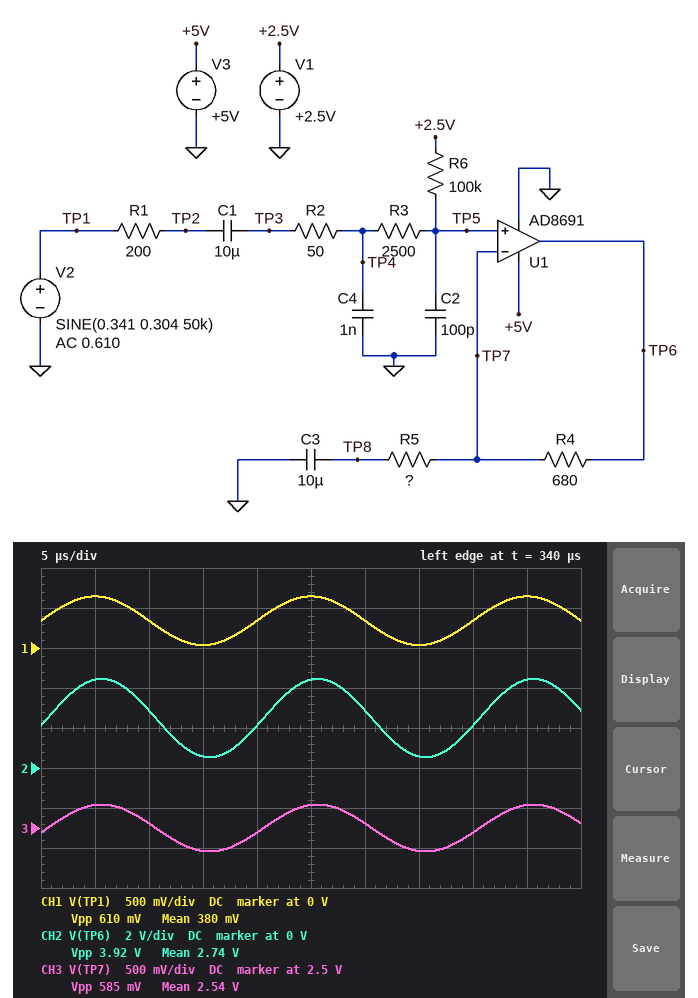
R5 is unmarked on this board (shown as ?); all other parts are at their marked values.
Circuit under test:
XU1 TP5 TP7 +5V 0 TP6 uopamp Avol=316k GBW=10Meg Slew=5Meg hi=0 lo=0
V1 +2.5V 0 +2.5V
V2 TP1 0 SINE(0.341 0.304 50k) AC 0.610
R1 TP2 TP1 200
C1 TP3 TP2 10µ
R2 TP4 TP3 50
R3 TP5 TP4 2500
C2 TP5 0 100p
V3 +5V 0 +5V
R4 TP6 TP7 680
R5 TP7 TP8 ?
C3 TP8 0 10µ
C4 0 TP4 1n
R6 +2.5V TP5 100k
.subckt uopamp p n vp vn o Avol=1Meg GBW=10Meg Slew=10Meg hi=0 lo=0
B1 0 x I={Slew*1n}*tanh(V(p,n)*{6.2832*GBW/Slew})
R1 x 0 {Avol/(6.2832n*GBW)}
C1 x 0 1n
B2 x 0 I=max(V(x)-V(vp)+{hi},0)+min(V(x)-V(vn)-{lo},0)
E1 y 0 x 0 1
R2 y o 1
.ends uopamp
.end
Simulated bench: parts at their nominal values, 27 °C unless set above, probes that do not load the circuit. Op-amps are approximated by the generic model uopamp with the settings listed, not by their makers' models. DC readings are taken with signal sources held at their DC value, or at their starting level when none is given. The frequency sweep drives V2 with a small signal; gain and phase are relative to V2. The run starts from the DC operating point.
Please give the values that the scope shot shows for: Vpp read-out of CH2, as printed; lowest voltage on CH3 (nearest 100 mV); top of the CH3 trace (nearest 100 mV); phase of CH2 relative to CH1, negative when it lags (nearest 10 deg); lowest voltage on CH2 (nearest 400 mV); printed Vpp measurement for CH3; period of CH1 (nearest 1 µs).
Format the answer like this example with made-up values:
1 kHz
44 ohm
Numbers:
3.92 V
2.2 V
2.8 V
-10 deg
400 mV
585 mV
20 µs
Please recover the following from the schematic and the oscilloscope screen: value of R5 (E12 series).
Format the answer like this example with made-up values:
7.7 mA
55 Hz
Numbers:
120 Ω
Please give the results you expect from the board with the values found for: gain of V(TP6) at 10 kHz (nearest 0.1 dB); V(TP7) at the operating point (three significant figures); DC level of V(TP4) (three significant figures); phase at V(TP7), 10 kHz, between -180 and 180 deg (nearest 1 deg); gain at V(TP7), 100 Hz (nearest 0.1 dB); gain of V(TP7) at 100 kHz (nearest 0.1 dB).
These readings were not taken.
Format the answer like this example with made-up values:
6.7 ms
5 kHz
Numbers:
16.2 dB
2.50 V
2.50 V
-2 deg
-0.2 dB
-0.5 dB
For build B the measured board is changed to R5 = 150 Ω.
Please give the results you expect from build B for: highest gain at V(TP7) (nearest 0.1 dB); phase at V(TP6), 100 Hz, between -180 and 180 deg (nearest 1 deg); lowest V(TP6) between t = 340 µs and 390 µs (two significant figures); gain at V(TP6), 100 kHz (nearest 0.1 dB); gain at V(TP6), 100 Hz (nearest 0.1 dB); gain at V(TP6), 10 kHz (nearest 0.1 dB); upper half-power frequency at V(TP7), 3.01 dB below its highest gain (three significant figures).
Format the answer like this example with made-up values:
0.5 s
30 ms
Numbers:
-0.2 dB
36 deg
870 mV
14.4 dB
11.5 dB
14.6 dB
374 kHz
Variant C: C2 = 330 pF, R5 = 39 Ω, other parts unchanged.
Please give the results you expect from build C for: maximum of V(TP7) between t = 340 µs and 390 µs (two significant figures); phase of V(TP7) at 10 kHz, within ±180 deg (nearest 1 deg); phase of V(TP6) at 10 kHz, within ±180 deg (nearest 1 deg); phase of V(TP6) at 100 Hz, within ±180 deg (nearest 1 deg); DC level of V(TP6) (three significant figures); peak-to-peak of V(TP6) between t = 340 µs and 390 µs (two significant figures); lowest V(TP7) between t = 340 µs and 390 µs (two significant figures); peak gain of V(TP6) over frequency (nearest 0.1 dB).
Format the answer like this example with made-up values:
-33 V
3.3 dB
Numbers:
2.6 V
-5 deg
-3 deg
64 deg
2.50 V
5.0 V
2.4 V
25.1 dB
